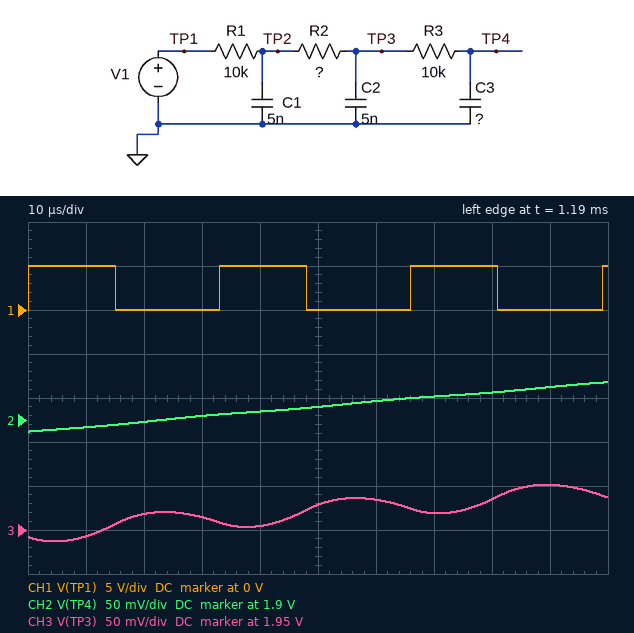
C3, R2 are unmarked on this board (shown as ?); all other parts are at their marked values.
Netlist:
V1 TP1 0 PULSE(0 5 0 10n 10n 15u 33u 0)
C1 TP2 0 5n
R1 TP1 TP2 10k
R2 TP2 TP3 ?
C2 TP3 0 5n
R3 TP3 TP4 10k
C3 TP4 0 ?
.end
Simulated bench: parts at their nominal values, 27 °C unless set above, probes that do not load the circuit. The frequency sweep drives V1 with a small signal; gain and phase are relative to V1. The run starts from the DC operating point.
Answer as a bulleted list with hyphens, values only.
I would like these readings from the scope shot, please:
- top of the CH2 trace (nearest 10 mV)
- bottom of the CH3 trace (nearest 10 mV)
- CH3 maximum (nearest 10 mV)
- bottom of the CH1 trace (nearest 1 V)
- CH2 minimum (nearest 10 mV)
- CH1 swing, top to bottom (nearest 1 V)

- 1.94 V
- 1.94 V
- 2.00 V
- 0 V
- 1.89 V
- 5 V
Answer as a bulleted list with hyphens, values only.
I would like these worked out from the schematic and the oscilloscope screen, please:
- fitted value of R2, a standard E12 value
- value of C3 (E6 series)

- 27 kΩ
- 10 nF
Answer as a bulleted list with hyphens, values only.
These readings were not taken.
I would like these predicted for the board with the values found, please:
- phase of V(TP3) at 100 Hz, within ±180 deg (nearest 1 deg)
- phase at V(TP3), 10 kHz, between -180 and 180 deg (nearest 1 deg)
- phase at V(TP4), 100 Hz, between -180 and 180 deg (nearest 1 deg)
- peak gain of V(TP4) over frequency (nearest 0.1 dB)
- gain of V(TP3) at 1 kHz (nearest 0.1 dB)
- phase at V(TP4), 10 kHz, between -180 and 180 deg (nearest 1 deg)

- -21 deg
- -135 deg
- -24 deg
- 0 dB
- -11.3 dB
- 144 deg
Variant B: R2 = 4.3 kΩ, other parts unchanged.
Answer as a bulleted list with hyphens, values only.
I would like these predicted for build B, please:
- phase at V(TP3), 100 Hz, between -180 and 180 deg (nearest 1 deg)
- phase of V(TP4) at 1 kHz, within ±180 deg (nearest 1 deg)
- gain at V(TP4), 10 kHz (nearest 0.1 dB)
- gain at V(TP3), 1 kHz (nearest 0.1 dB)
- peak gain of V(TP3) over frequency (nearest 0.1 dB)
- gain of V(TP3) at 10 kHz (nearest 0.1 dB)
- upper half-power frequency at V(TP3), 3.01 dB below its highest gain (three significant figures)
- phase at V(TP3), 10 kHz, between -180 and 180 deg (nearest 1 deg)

- -9 deg
- -80 deg
- -35.5 dB
- -5.8 dB
- 0 dB
- -19.5 dB
- 549 Hz
- -103 deg
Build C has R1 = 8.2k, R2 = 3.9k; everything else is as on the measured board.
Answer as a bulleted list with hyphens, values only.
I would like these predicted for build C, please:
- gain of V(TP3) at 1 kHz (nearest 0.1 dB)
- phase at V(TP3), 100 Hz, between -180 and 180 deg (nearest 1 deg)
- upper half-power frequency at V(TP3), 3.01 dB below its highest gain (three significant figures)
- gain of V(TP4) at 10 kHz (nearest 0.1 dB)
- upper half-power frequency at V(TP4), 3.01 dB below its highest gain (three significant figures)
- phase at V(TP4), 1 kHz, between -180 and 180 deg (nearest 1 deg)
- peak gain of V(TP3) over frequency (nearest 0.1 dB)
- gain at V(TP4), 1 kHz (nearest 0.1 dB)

- -4.9 dB
- -8 deg
- 646 Hz
- -33.7 dB
- 562 Hz
- -76 deg
- 0 dB
- -6.3 dB
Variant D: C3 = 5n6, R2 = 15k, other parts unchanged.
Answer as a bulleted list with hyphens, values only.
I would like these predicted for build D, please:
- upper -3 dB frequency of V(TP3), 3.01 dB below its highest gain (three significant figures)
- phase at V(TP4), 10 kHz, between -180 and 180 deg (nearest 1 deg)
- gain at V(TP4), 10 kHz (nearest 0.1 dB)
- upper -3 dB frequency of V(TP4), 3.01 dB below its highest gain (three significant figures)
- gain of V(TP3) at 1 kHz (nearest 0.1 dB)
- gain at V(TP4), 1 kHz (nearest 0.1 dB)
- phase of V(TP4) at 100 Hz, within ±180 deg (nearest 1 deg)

- 510 Hz
- 157 deg
- -37.5 dB
- 494 Hz
- -6.7 dB
- -7.2 dB
- -13 deg
